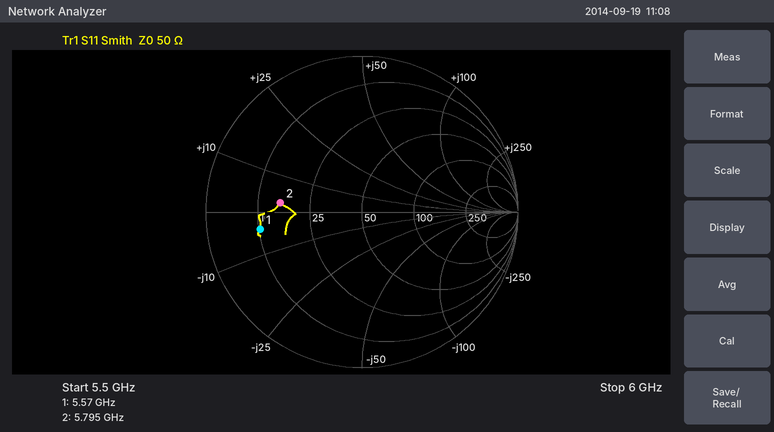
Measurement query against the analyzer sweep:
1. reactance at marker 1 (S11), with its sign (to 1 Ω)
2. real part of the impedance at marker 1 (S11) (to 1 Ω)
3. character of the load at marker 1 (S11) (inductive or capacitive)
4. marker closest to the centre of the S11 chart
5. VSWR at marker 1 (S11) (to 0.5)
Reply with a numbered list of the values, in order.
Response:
1. -4 Ω
2. 10 Ω
3. capacitive
4. marker 2
5. 5.0
